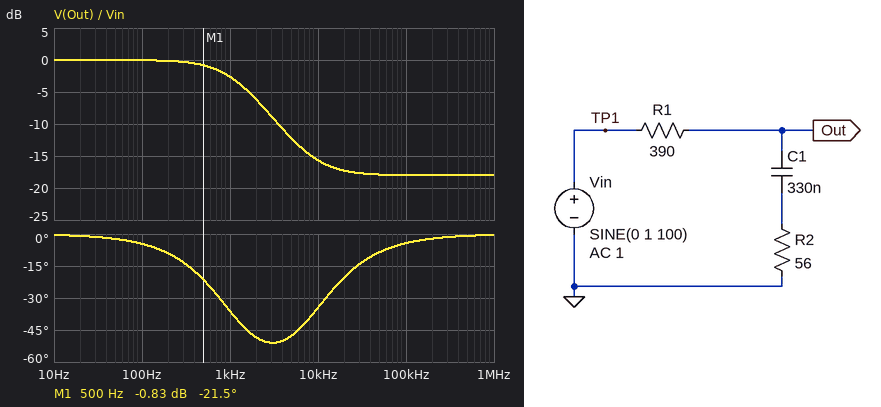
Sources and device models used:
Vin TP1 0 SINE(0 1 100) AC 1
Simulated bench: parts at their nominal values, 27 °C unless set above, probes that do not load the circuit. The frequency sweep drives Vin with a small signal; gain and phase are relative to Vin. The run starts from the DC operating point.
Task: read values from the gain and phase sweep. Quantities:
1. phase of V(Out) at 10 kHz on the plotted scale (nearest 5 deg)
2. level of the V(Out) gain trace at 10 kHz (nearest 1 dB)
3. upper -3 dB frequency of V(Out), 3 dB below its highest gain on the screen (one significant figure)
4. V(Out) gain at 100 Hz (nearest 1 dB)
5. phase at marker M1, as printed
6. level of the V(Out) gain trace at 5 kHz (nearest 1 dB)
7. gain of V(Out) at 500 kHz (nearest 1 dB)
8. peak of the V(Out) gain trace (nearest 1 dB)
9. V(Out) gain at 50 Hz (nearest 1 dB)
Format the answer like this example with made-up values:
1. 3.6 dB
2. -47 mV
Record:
1. -35 deg
2. -16 dB
3. 1 kHz
4. 0 dB
5. -21.5 deg
6. -12 dB
7. -18 dB
8. 0 dB
9. 0 dB
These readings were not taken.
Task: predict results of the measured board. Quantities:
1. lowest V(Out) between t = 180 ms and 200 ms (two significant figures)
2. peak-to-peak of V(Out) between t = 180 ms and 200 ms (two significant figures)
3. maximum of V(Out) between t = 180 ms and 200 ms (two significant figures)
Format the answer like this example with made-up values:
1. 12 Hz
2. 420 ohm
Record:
1. -1.0 V
2. 2.0 V
3. 1.0 V
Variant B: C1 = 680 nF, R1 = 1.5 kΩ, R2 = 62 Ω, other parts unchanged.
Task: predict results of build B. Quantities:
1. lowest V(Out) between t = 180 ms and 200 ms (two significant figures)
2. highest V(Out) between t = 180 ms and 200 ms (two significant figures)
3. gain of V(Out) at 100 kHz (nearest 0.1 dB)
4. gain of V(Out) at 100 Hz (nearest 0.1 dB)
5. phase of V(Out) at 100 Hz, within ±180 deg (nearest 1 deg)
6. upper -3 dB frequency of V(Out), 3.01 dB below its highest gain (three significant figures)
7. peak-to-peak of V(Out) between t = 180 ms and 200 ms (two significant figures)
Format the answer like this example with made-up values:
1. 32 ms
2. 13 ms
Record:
1. -830 mV
2. 830 mV
3. -28.0 dB
4. -1.6 dB
5. -32 deg
6. 150 Hz
7. 1.7 V
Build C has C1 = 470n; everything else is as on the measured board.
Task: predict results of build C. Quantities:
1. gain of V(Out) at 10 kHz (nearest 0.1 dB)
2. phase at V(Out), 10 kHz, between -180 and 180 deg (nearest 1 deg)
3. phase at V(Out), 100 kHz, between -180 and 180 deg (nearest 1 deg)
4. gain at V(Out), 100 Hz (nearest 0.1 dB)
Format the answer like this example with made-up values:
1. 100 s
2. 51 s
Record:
1. -16.7 dB
2. -27 deg
3. -3 deg
4. -0.1 dB
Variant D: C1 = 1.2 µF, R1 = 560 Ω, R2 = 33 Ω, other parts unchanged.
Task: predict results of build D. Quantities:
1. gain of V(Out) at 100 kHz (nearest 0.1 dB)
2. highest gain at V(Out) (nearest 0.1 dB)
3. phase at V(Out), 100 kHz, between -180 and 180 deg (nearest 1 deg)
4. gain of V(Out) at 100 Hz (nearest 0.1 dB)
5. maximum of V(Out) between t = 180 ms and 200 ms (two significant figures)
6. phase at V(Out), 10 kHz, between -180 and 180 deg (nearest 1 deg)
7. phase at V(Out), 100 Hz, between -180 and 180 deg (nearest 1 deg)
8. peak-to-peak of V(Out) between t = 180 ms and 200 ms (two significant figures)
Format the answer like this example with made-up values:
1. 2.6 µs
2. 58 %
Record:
1. -25.1 dB
2. 0 dB
3. -2 deg
4. -0.8 dB
5. 910 mV
6. -21 deg
7. -23 deg
8. 1.8 V
